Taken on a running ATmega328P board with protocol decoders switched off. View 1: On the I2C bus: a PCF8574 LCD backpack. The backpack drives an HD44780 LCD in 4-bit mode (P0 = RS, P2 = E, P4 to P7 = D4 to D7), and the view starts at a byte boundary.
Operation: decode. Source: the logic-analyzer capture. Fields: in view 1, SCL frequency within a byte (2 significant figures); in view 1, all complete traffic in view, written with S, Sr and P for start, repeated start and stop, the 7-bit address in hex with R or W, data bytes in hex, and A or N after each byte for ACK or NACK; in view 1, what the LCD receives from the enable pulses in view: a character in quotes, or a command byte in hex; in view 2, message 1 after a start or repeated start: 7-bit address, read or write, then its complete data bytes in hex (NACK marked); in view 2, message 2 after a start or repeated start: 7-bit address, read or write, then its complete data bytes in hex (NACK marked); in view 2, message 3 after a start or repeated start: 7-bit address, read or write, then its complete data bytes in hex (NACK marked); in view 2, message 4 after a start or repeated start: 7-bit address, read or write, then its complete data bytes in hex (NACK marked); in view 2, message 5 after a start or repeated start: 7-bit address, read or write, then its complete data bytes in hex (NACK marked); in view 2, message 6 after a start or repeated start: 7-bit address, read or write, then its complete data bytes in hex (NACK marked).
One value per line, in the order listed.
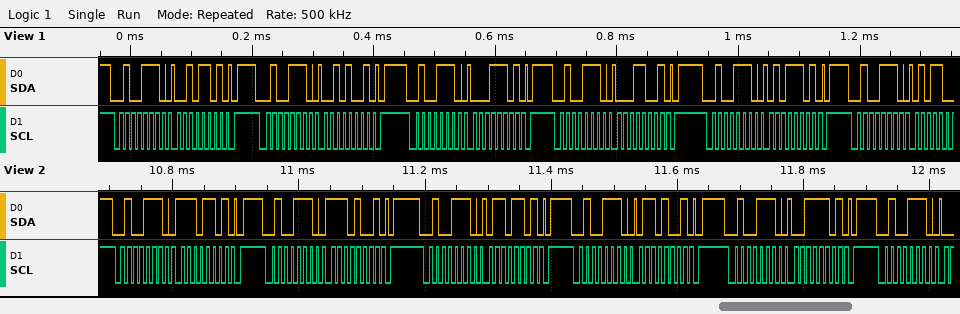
100 kHz
S 27W A 2D A P S 27W A 29 A P S 27W A 1D A P S 27W A 19 A P S 27W A 5D A P S 27W A
'!'
0x27 write: ED
0x27 write: E9
0x27 write: 6D
0x27 write: 69
0x27 write: 3D
0x27 write
